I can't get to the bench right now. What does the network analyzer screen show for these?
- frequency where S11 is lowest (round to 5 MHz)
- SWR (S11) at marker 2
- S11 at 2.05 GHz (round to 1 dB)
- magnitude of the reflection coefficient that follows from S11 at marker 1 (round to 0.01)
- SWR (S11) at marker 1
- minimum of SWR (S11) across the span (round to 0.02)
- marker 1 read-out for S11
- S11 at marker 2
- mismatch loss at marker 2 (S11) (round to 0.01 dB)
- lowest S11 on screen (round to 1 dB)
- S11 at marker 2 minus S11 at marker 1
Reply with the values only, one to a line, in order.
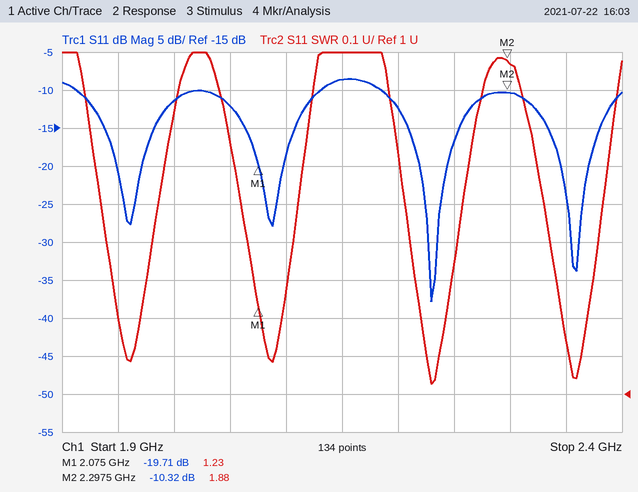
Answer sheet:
2.230 GHz
1.88
-12 dB
0.10
1.23
1.02
-19.71 dB
-10.32 dB
0.42 dB
-38 dB
9.39 dB
